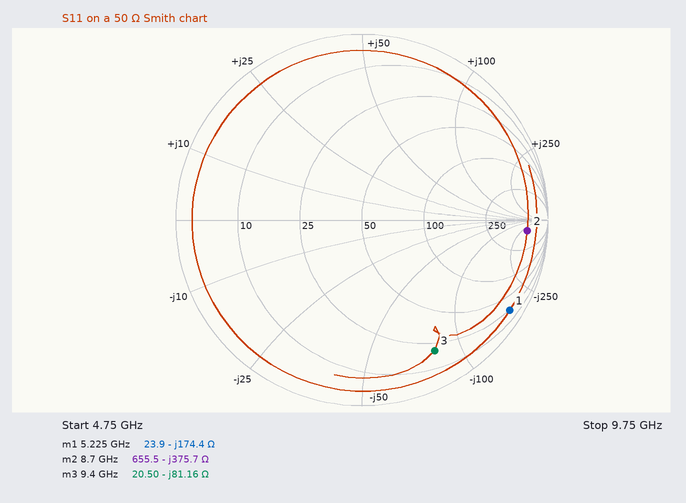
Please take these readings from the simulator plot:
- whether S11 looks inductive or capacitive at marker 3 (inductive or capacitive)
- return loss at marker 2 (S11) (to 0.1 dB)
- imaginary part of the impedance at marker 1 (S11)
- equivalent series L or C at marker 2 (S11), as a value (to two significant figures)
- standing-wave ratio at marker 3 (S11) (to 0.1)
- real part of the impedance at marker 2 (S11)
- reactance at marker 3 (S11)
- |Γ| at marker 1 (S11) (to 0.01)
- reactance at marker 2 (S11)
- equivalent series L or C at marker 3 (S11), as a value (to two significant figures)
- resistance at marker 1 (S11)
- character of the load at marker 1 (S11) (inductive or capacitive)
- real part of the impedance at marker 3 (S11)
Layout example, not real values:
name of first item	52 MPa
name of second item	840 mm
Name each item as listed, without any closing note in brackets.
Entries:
whether S11 looks inductive or capacitive at marker 3	capacitive
return loss at marker 2 (S11)	1.0 dB
imaginary part of the impedance at marker 1	-174.4 Ω
equivalent series L or C at marker 2 (S11), as a value	49 fF
standing-wave ratio at marker 3 (S11)	9.2
real part of the impedance at marker 2	655.5 Ω
reactance at marker 3	-81.16 Ω
|Γ| at marker 1 (S11)	0.93
reactance at marker 2	-375.7 Ω
equivalent series L or C at marker 3 (S11), as a value	210 fF
resistance at marker 1	23.9 Ω
character of the load at marker 1 (S11)	capacitive
real part of the impedance at marker 3	20.50 Ω
